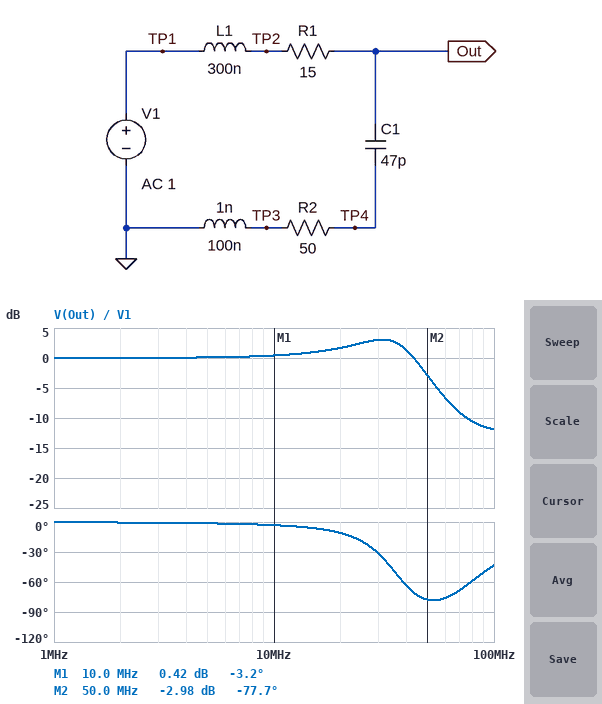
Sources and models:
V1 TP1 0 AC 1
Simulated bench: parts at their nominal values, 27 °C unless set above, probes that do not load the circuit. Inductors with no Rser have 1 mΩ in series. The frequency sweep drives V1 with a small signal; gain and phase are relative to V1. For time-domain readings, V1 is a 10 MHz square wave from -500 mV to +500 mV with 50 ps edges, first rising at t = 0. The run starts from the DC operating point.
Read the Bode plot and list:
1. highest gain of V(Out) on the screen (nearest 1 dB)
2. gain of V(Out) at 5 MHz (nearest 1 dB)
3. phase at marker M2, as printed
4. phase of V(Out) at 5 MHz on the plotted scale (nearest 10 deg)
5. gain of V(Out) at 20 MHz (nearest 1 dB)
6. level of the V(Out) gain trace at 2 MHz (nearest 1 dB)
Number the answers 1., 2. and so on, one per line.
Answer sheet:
1. 3 dB
2. 0 dB
3. -77.7 deg
4. 0 deg
5. 2 dB
6. 0 dB
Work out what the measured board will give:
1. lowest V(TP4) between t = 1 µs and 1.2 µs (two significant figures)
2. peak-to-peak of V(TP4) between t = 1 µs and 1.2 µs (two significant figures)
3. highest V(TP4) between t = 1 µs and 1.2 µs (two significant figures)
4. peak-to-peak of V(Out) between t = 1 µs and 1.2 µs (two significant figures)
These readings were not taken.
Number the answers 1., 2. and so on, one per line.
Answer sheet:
1. -390 mV
2. 780 mV
3. 390 mV
4. 1.5 V
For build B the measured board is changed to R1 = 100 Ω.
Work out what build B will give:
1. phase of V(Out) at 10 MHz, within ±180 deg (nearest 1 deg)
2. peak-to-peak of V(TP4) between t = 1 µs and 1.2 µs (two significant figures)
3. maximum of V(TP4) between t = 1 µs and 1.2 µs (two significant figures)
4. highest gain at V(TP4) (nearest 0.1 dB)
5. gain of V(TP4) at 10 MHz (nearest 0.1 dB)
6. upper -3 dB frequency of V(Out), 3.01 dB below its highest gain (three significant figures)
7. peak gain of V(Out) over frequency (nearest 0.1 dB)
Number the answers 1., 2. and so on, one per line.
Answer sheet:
1. -17 deg
2. 550 mV
3. 270 mV
4. -8.6 dB
5. -16.8 dB
6. 29.0 MHz
7. 0 dB
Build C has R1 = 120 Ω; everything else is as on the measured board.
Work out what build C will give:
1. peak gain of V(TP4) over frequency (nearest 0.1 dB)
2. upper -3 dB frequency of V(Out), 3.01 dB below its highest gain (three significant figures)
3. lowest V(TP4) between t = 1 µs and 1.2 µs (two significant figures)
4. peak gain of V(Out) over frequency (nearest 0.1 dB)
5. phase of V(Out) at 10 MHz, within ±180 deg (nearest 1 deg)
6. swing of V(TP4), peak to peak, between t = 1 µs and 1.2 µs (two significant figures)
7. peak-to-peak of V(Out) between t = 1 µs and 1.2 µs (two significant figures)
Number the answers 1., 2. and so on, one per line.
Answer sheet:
1. -9.6 dB
2. 24.7 MHz
3. -260 mV
4. 0 dB
5. -20 deg
6. 520 mV
7. 1.0 V
